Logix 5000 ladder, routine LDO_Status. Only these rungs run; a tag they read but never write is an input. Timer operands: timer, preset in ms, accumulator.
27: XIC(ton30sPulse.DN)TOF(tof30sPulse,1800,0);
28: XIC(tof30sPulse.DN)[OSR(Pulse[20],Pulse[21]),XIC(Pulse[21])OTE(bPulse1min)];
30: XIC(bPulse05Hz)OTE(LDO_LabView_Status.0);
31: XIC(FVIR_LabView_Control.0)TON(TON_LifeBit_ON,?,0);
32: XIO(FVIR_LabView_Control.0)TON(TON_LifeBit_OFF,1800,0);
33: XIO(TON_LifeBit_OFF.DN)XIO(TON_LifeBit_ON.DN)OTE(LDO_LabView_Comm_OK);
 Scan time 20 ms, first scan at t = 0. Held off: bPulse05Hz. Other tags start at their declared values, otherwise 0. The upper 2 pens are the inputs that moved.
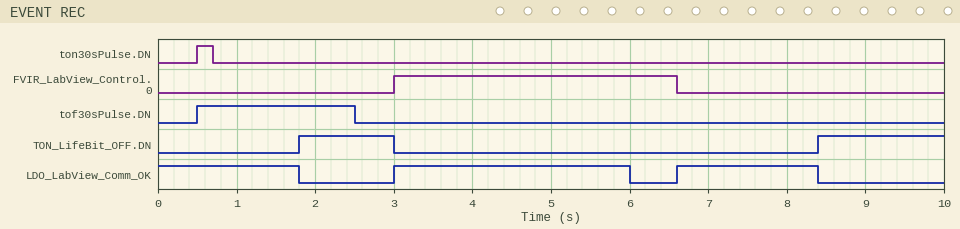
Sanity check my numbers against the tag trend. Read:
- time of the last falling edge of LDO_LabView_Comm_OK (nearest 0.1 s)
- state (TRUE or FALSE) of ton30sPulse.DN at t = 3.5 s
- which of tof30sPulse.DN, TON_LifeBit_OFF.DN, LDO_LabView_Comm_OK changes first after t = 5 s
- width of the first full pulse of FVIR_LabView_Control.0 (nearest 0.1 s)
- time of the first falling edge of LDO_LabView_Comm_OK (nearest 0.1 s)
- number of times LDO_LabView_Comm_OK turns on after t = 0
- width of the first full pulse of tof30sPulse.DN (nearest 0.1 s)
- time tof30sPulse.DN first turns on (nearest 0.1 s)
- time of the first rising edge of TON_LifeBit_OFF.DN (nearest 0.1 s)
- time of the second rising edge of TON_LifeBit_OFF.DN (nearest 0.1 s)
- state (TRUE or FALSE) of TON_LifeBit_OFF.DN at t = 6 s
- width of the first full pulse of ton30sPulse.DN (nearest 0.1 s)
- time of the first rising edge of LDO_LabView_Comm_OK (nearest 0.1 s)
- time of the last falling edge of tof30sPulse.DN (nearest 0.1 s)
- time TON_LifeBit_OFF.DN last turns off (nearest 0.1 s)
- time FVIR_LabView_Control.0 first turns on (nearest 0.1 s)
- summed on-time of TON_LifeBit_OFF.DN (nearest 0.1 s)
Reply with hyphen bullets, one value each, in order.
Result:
- 8.4 s
- FALSE
- LDO_LabView_Comm_OK
- 3.6 s
- 1.8 s
- 2
- 2.0 s
- 0.5 s
- 1.8 s
- 8.4 s
- FALSE
- 0.2 s
- 3.0 s
- 2.5 s
- 3.0 s
- 3.0 s
- 2.8 s
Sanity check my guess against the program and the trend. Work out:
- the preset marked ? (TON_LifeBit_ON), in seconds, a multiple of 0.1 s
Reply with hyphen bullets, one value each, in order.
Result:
- 3.0 s
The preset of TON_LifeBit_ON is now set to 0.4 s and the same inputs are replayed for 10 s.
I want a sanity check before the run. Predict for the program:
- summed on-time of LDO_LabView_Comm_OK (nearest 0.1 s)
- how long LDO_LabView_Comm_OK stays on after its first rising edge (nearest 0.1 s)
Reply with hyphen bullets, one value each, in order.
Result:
- 4.0 s
- 0.4 s
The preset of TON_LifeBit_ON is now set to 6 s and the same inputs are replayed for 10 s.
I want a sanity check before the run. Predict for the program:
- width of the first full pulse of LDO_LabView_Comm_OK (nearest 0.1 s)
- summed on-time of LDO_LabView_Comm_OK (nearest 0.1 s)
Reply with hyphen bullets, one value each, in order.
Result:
- 5.4 s
- 7.2 s
